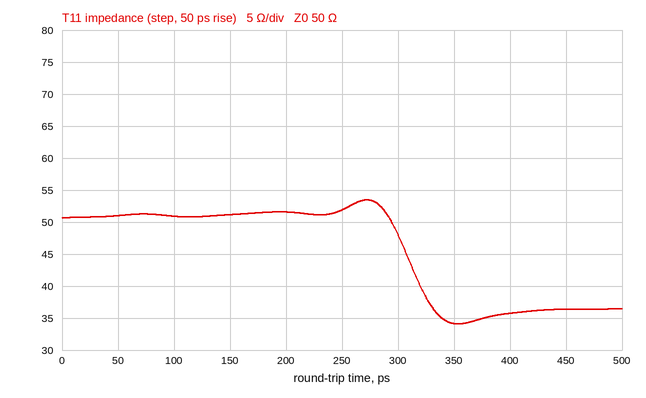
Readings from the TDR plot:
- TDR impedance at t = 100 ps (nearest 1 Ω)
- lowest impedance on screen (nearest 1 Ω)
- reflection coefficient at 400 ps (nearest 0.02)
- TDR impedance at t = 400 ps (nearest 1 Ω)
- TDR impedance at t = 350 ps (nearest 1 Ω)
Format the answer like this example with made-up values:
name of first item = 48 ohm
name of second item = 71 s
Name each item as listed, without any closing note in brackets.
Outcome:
TDR impedance at t = 100 ps = 51 Ω
lowest impedance on screen = 34 Ω
reflection coefficient at 400 ps = -0.16
TDR impedance at t = 400 ps = 36 Ω
TDR impedance at t = 350 ps = 34 Ω
